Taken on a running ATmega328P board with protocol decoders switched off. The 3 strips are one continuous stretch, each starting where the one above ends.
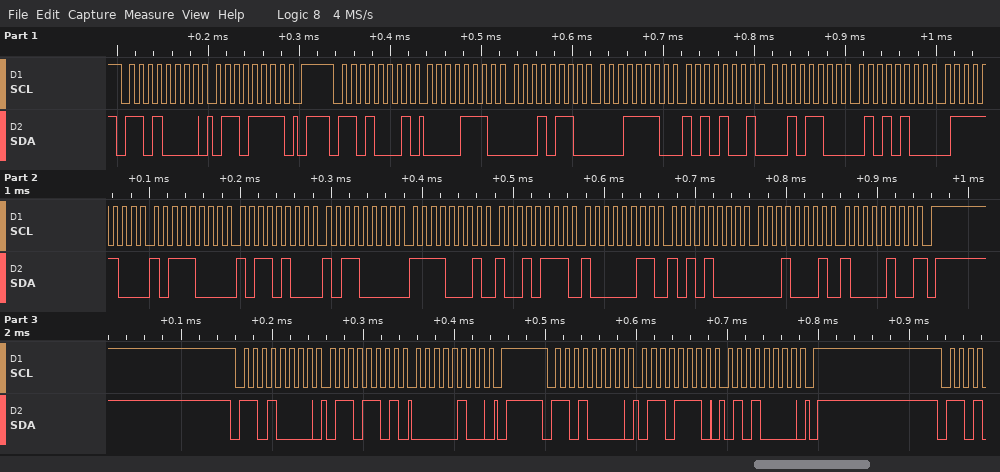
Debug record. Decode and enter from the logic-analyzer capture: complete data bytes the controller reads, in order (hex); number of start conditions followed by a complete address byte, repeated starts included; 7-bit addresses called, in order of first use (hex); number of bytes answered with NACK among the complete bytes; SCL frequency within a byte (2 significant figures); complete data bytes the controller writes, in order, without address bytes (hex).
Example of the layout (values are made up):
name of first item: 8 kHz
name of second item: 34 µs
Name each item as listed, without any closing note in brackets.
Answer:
complete data bytes the controller reads, in order: 0E 16 1E A9 2C 54 7C B8 B4 B0 F1 97 83 A8 11 84
number of start conditions followed by a complete address byte, repeated starts included: 4
7-bit addresses called, in order of first use: 0x68
number of bytes answered with NACK among the complete bytes: 1
SCL frequency within a byte: 100 kHz
complete data bytes the controller writes, in order, without address bytes: 6F 6D 04 6E 50
